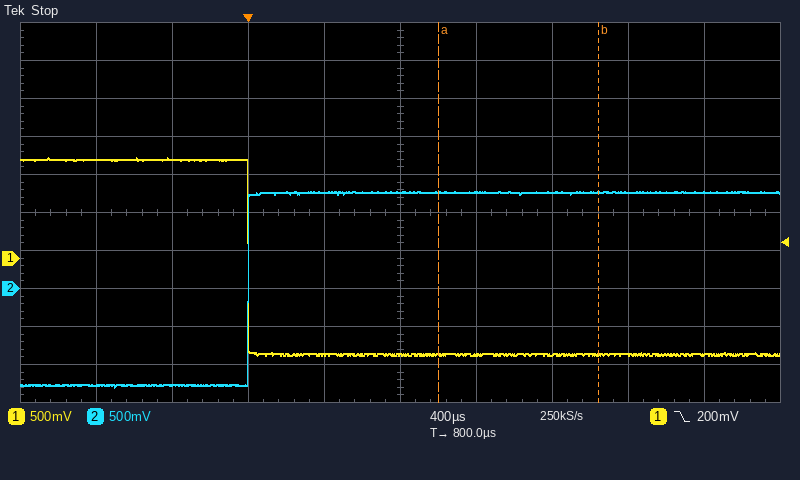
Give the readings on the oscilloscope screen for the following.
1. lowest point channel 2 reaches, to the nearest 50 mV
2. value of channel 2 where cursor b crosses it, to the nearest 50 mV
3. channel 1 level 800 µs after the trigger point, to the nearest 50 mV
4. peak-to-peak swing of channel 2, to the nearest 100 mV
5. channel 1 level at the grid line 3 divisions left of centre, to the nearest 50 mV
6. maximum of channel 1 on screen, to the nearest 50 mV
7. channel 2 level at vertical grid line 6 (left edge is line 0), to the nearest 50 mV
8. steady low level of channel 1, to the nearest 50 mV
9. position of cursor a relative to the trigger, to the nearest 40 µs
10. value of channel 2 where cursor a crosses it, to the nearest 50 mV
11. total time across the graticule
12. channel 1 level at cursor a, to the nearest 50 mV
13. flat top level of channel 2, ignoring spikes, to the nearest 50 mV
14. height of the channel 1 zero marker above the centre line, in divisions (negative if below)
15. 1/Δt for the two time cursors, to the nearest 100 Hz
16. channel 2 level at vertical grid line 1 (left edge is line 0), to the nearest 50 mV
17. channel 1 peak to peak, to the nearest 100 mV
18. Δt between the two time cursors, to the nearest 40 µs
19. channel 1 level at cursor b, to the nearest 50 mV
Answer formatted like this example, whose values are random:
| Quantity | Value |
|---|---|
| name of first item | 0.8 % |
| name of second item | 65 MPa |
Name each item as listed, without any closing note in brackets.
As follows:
| Quantity | Value |
|---|---|
| lowest point channel 2 reaches, to the nearest 50 mV | -1.30 V |
| value of channel 2 where cursor b crosses it, to the nearest 50 mV | 1.25 V |
| channel 1 level 800 µs after the trigger point, to the nearest 50 mV | -1.25 V |
| peak-to-peak swing of channel 2, to the nearest 100 mV | 2.60 V |
| channel 1 level at the grid line 3 divisions left of centre, to the nearest 50 mV | 1.30 V |
| maximum of channel 1 on screen, to the nearest 50 mV | 1.30 V |
| channel 2 level at vertical grid line 6 (left edge is line 0), to the nearest 50 mV | 1.25 V |
| steady low level of channel 1, to the nearest 50 mV | -1.25 V |
| position of cursor a relative to the trigger, to the nearest 40 µs | +1.00 ms |
| value of channel 2 where cursor a crosses it, to the nearest 50 mV | 1.25 V |
| total time across the graticule | 4 ms |
| channel 1 level at cursor a, to the nearest 50 mV | -1.25 V |
| flat top level of channel 2, ignoring spikes, to the nearest 50 mV | 1.25 V |
| height of the channel 1 zero marker above the centre line, in divisions | -1.2 div |
| 1/Δt for the two time cursors, to the nearest 100 Hz | 1.2 kHz |
| channel 2 level at vertical grid line 1 (left edge is line 0), to the nearest 50 mV | -1.25 V |
| channel 1 peak to peak, to the nearest 100 mV | 2.60 V |
| Δt between the two time cursors, to the nearest 40 µs | 840 µs |
| channel 1 level at cursor b, to the nearest 50 mV | -1.25 V |
